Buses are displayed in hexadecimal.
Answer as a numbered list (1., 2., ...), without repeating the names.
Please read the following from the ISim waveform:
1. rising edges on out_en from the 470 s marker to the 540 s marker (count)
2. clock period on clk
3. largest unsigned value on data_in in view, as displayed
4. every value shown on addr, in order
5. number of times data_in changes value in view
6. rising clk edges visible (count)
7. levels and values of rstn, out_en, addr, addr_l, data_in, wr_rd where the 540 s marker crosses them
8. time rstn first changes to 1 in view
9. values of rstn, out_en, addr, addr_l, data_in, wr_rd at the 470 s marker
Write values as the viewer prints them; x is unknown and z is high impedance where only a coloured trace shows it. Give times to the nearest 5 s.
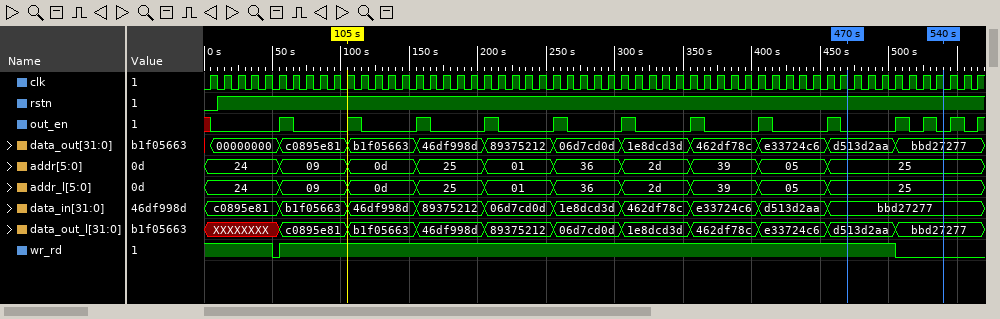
1. 2
2. 10 s
3. e33724c6
4. 24, 09, 0d, 25, 01, 36, 2d, 39, 05, 25
5. 9
6. 57
7. rstn=1, out_en=0, addr=25, addr_l=25, data_in=bbd27277, wr_rd=0
8. 10 s
9. rstn=1, out_en=0, addr=25, addr_l=25, data_in=bbd27277, wr_rd=1
